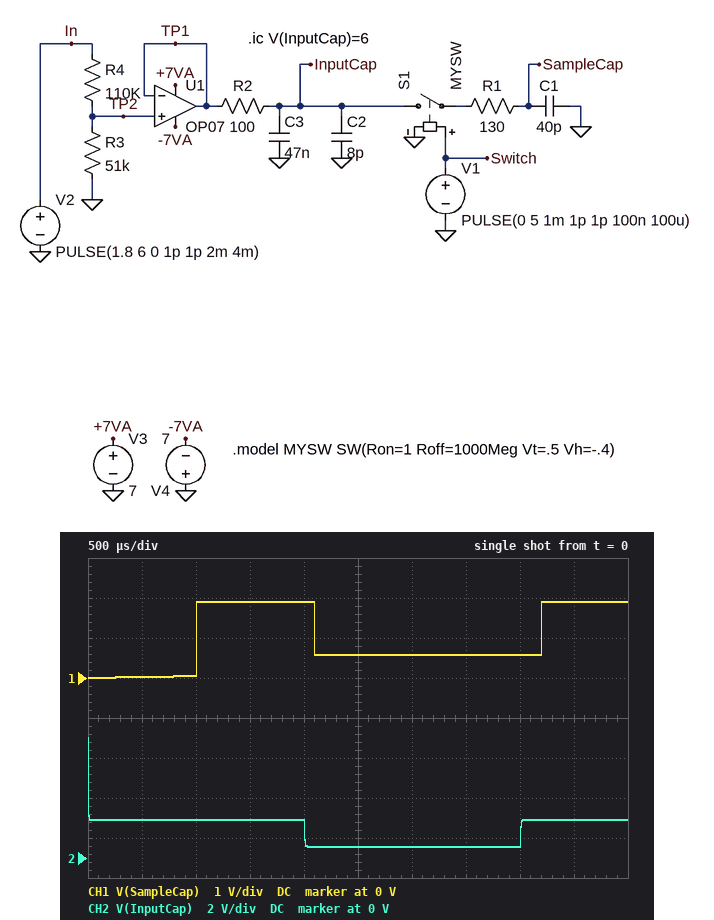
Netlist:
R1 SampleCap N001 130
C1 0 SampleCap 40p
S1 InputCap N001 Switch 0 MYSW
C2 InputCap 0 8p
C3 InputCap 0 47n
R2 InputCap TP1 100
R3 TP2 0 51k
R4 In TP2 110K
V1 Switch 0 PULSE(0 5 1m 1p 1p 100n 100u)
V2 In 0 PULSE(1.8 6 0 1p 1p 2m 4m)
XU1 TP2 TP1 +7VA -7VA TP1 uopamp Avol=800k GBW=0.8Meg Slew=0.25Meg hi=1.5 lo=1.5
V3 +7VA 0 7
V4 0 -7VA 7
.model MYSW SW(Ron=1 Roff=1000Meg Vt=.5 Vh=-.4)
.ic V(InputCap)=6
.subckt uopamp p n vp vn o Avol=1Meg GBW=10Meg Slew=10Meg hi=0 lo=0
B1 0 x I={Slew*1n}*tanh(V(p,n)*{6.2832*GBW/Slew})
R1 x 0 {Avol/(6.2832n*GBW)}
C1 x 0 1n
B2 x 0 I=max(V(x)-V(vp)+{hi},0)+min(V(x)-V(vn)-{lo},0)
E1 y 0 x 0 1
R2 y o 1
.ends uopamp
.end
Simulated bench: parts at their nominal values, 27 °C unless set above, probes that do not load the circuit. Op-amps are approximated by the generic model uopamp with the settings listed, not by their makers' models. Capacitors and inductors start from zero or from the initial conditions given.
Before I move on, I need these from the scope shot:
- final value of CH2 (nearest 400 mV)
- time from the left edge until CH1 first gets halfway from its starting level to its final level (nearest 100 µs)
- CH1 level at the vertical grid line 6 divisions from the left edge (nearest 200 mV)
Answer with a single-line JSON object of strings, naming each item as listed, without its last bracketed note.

{"final value of CH2": "2.0 V", "time from the left edge until CH1 first gets halfway from its starting level to its final level": "1.0 ms", "CH1 level at the vertical grid line 6 divisions from the left edge": "600 mV"}
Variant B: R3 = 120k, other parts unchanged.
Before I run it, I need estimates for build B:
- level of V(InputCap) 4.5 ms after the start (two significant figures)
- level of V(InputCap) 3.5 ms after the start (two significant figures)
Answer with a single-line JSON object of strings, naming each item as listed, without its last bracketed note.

{"level of V(InputCap) 4.5 ms after the start": "3.1 V", "level of V(InputCap) 3.5 ms after the start": "940 mV"}
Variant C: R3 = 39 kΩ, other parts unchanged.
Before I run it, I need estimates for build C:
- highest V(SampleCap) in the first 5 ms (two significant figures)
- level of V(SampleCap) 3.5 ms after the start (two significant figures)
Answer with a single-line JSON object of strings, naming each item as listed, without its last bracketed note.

{"highest V(SampleCap) in the first 5 ms": "1.6 V", "level of V(SampleCap) 3.5 ms after the start": "470 mV"}
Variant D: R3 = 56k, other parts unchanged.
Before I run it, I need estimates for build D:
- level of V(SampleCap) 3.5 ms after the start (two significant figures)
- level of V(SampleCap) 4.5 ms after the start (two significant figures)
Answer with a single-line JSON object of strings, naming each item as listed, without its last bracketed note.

{"level of V(SampleCap) 3.5 ms after the start": "610 mV", "level of V(SampleCap) 4.5 ms after the start": "2.0 V"}
